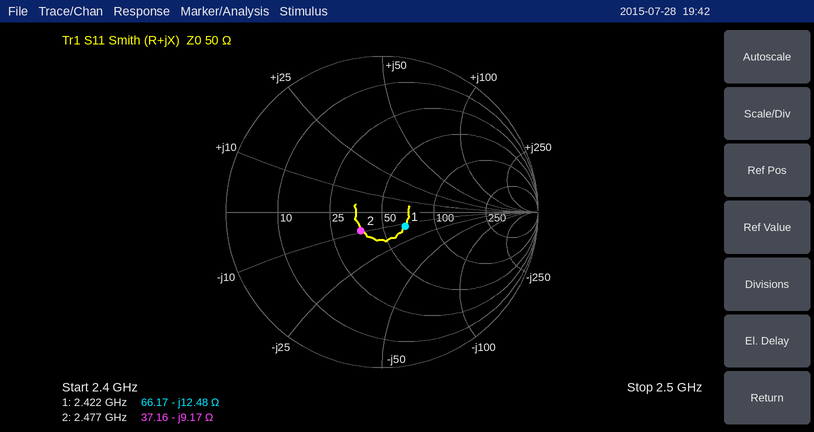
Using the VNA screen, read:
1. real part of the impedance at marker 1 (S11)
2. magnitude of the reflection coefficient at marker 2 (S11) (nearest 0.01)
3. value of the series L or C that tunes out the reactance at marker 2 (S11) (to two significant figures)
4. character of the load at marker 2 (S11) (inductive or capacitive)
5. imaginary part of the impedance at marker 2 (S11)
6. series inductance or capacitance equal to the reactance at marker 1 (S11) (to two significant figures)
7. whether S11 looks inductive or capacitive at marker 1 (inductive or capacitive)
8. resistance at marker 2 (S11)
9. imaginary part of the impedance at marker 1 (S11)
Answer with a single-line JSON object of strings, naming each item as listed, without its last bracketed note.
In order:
{"real part of the impedance at marker 1": "66.17 Ω", "magnitude of the reflection coefficient at marker 2 (S11)": "0.18", "value of the series L or C that tunes out the reactance at marker 2 (S11)": "590 pH", "character of the load at marker 2 (S11)": "capacitive", "imaginary part of the impedance at marker 2": "-9.17 Ω", "series inductance or capacitance equal to the reactance at marker 1 (S11)": "5.3 pF", "whether S11 looks inductive or capacitive at marker 1": "capacitive", "resistance at marker 2": "37.16 Ω", "imaginary part of the impedance at marker 1": "-12.48 Ω"}
